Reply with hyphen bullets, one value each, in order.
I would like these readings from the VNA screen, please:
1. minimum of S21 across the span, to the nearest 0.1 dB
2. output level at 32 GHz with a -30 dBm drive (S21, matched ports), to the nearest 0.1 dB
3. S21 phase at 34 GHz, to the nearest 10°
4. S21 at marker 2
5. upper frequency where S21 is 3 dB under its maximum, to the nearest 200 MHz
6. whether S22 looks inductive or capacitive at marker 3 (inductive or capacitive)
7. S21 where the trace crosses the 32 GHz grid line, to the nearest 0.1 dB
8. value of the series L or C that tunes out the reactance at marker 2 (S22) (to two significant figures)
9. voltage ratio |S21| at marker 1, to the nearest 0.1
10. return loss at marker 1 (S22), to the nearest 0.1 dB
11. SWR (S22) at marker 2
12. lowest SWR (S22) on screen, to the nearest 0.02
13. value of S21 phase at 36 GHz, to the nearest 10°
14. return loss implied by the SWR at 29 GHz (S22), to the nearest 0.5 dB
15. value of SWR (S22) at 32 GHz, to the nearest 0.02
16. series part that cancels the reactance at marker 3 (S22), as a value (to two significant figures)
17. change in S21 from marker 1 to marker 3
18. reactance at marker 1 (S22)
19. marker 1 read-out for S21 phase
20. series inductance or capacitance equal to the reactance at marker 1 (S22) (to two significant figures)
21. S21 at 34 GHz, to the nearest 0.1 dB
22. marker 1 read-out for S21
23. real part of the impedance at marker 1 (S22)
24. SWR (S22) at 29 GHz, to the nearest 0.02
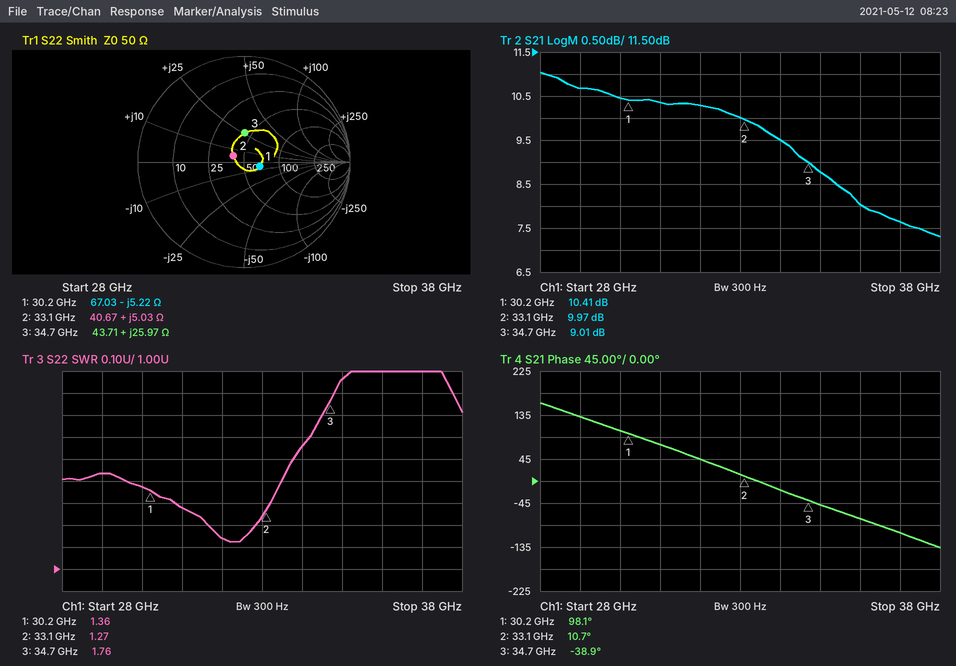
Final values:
- 7.3 dB
- -19.7 dBm
- -20°
- 9.97 dB
- 36.0 GHz
- inductive
- 10.3 dB
- 960 fF
- 3.3
- 16.4 dB
- 1.27
- 1.12
- -80°
- 15.0 dB
- 1.14
- 180 fF
- -1.40 dB
- -5.22 Ω
- 98.1°
- 1.0 pF
- 9.5 dB
- 10.41 dB
- 67.03 Ω
- 1.44
